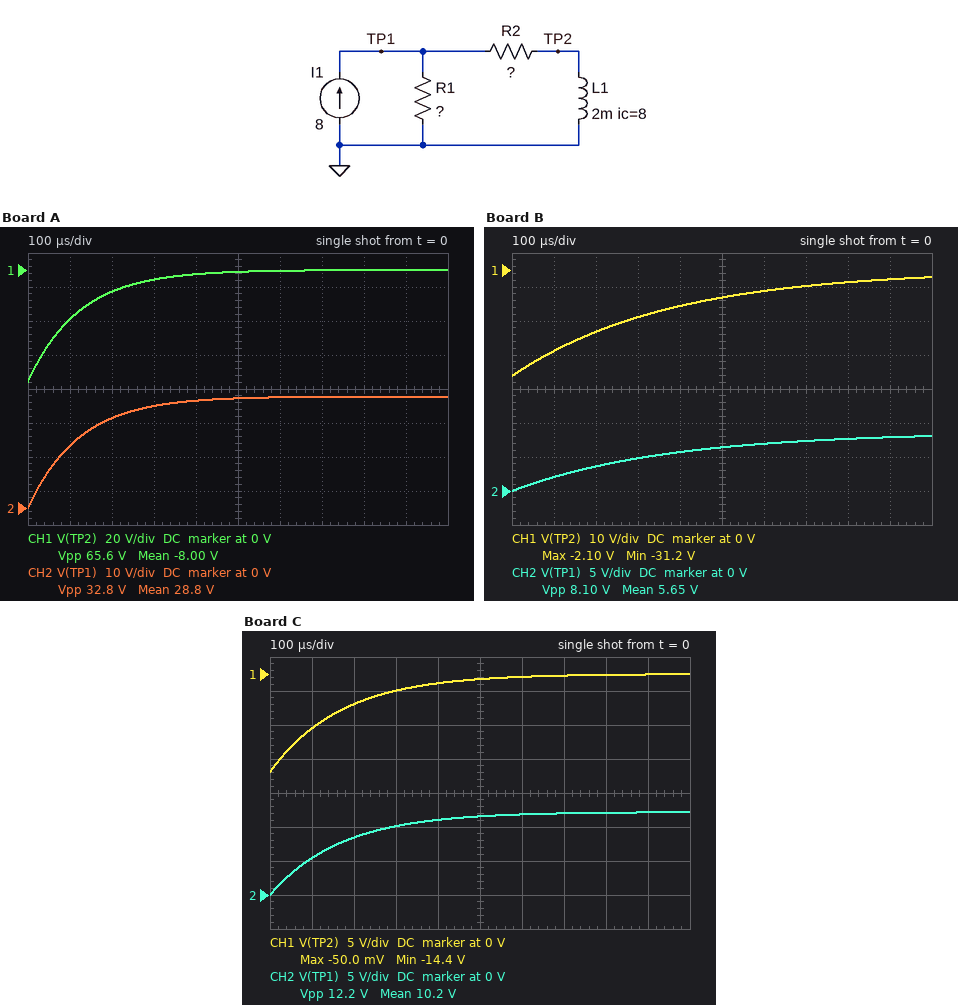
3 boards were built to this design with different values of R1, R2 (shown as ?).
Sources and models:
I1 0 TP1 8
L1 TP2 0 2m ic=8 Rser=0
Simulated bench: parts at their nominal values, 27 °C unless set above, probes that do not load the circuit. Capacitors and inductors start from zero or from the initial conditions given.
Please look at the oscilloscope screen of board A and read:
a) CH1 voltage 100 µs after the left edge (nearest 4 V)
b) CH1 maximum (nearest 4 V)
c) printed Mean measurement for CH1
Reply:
-28 V
0 V
-8.00 V
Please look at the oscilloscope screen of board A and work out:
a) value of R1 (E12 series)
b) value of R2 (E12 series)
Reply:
8.2 Ω
8.2 Ω
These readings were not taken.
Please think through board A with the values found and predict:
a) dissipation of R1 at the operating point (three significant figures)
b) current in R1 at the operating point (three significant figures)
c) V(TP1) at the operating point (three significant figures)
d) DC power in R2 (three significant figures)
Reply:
131 W
4.00 A
32.8 V
131 W
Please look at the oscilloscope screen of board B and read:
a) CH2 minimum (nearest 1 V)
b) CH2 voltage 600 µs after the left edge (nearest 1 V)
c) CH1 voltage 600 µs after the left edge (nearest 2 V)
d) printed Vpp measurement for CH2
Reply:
0 V
7 V
-6 V
8.10 V
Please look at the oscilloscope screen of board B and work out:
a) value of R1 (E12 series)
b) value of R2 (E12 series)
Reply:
1.5 Ω
3.9 Ω
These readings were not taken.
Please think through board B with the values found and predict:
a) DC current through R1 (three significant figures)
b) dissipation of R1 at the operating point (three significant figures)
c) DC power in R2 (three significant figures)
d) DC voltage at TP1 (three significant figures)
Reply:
5.78 A
50.1 W
19.3 W
8.67 V
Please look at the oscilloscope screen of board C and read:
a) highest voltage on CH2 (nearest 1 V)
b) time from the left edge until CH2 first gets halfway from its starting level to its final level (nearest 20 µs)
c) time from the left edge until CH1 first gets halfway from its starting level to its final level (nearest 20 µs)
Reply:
12 V
120 µs
120 µs
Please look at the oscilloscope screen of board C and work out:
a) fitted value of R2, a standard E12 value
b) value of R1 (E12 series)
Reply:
1.8 Ω
10 Ω
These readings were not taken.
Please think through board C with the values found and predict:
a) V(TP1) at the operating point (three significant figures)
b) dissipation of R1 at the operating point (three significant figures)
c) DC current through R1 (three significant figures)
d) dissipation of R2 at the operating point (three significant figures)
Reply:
12.2 V
14.9 W
1.22 A
82.7 W
